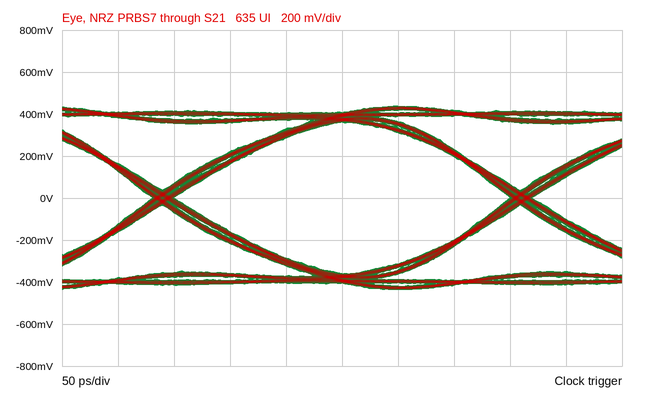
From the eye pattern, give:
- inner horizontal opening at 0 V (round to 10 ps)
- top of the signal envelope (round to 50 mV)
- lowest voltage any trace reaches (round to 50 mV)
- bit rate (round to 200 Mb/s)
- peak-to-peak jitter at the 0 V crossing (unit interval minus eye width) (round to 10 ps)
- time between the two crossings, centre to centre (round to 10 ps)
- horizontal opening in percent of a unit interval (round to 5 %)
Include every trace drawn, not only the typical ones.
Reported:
300 ps
450 mV
-450 mV
3.2 Gb/s
20 ps
320 ps
95 %
